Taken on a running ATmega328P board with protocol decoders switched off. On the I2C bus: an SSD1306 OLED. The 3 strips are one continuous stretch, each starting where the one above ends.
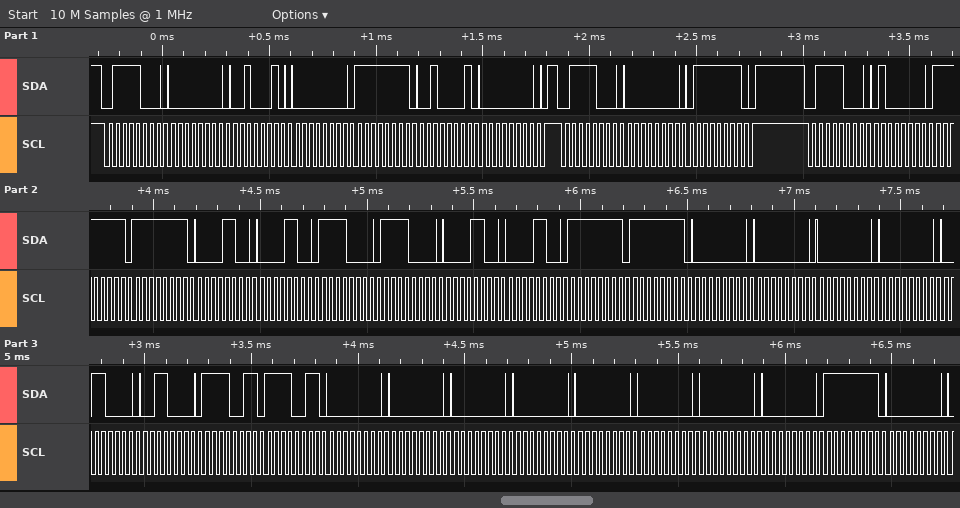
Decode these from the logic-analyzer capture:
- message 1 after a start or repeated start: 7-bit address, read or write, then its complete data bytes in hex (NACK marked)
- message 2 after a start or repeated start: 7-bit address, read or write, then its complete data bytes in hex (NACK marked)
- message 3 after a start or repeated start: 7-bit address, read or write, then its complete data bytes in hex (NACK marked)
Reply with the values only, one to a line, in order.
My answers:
0x3C write: 00 22 00 FF 21 00
0x3C write: 00 7F
0x3C write: 40 FF FF 0C 0C F0 F0 0C 0C FF FF 00 00 00 00 30 30 F3 F3 00 00 00 00 00 00 00 00 FF 00
